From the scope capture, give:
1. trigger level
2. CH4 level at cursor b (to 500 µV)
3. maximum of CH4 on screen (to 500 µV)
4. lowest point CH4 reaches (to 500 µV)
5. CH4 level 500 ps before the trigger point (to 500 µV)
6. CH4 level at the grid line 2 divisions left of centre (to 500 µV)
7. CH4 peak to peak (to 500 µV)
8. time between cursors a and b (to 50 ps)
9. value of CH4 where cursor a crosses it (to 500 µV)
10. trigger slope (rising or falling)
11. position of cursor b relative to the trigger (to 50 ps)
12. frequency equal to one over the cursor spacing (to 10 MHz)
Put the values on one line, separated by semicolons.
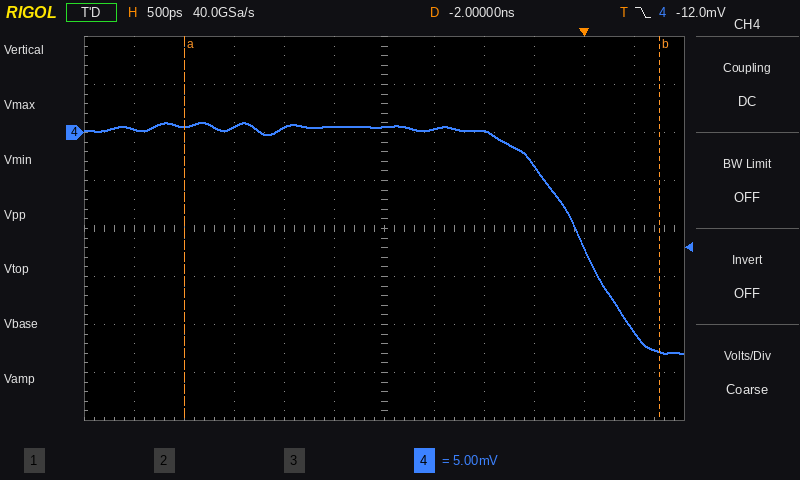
-12.0 mV; -23.0 mV; 1.0 mV; -23.0 mV; -3.5 mV; 500 µV; 24.0 mV; 4.75 ns; 500 µV; falling; +750 ps; 210 MHz
